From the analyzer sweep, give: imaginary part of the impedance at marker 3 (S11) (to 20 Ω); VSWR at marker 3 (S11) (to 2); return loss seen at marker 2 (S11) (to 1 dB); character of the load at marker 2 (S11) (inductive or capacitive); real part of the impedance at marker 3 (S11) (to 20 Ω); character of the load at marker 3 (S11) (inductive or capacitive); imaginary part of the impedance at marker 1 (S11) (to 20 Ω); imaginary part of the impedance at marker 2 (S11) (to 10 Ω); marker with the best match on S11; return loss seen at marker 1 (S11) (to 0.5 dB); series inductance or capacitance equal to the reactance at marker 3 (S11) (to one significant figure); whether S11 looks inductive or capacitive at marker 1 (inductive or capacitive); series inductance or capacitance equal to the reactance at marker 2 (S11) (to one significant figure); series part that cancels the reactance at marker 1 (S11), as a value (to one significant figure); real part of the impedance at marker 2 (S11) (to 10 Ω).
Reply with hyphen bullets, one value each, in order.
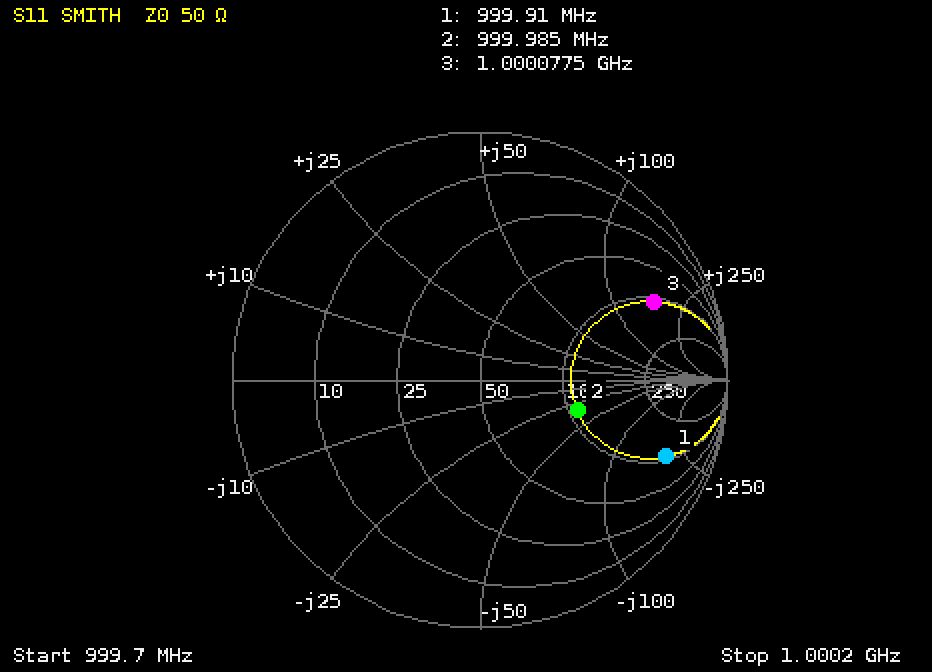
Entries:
- +160 Ω
- 8
- 8 dB
- capacitive
- 100 Ω
- inductive
- -200 Ω
- -30 Ω
- marker 2
- 2.0 dB
- 30 nH
- capacitive
- 5 pF
- 30 nH
- 110 Ω
